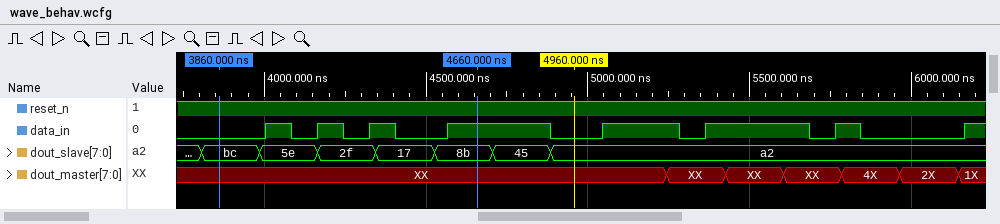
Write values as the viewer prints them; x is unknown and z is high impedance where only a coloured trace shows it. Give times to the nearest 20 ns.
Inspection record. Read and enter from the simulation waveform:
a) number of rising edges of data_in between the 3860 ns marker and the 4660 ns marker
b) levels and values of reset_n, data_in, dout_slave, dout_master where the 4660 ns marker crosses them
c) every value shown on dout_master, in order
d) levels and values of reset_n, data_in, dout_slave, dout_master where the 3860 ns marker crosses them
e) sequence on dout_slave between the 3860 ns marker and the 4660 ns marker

4
reset_n=1, data_in=1, dout_slave=8b, dout_master=XX
XX, XX, XX, XX, 4X, 2X, 1X
reset_n=1, data_in=0, dout_slave=bc, dout_master=XX
bc, 5e, 2f, 17, 8b
